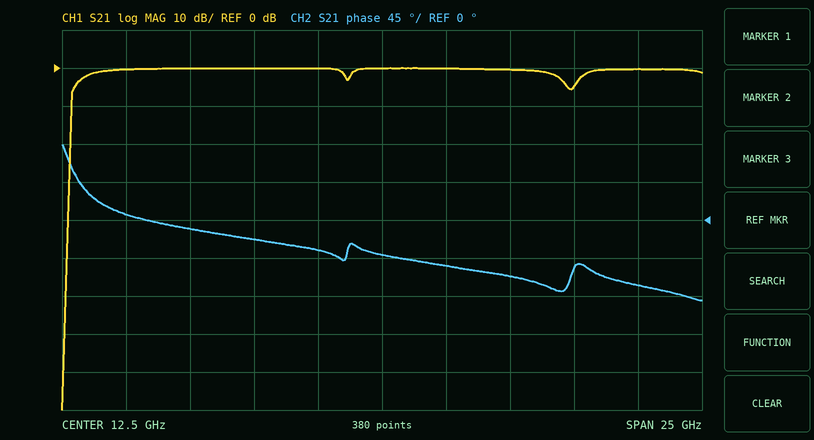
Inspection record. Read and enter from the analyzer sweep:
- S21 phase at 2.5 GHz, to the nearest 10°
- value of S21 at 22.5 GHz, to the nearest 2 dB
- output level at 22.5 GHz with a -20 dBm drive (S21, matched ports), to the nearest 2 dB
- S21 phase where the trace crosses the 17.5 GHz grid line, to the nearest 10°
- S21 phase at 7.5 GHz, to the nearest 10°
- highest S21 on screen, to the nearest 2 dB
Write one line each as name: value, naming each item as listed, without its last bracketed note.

S21 phase at 2.5 GHz, to the nearest 10°: 10°
value of S21 at 22.5 GHz, to the nearest 2 dB: 0 dB
output level at 22.5 GHz with a -20 dBm drive (S21, matched ports), to the nearest 2 dB: -20 dBm
S21 phase where the trace crosses the 17.5 GHz grid line, to the nearest 10°: -70°
S21 phase at 7.5 GHz, to the nearest 10°: -20°
highest S21 on screen, to the nearest 2 dB: 0 dB
